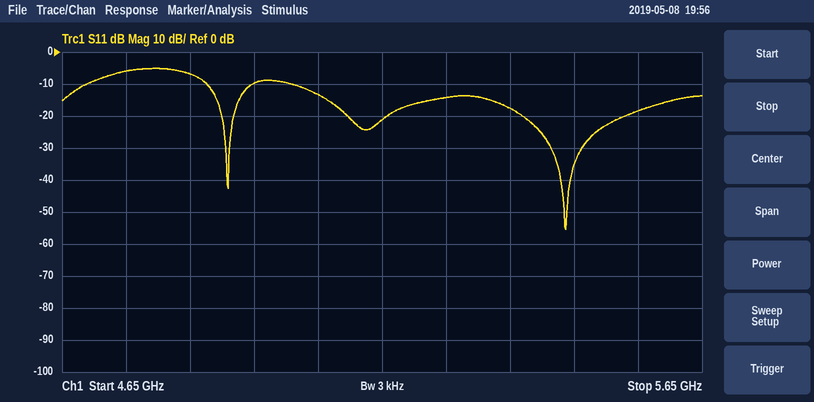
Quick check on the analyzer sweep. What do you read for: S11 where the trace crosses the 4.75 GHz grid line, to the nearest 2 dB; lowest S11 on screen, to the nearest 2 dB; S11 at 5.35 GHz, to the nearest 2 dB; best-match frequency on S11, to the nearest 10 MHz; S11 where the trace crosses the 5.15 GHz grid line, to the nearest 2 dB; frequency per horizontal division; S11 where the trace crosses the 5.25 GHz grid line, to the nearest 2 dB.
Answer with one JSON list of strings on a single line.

["-6 dB", "-56 dB", "-18 dB", "5.44 GHz", "-22 dB", "100 MHz", "-14 dB"]
